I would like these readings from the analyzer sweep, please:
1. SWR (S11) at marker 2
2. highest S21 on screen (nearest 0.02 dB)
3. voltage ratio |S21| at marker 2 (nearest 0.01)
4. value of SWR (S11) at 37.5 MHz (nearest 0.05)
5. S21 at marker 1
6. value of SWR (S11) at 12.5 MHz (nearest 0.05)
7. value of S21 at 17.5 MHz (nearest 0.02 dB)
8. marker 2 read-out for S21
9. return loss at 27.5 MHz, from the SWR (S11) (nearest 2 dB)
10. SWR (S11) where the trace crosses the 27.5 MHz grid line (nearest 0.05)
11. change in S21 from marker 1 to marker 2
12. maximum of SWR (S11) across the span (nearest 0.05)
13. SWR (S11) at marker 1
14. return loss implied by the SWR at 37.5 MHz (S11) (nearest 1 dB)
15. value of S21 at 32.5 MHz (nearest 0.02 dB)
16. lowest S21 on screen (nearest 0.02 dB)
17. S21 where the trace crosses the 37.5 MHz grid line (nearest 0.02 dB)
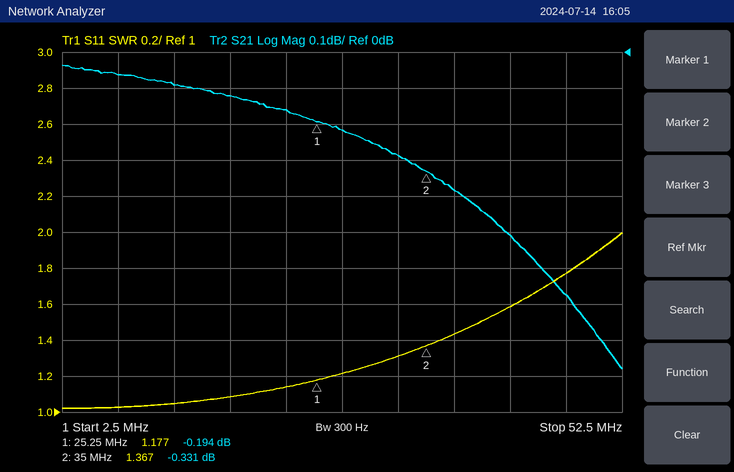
1.367
-0.04 dB
0.96
1.45
-0.194 dB
1.05
-0.12 dB
-0.331 dB
20 dB
1.20
-0.137 dB
2.00
1.177
15 dB
-0.28 dB
-0.88 dB
-0.38 dB
